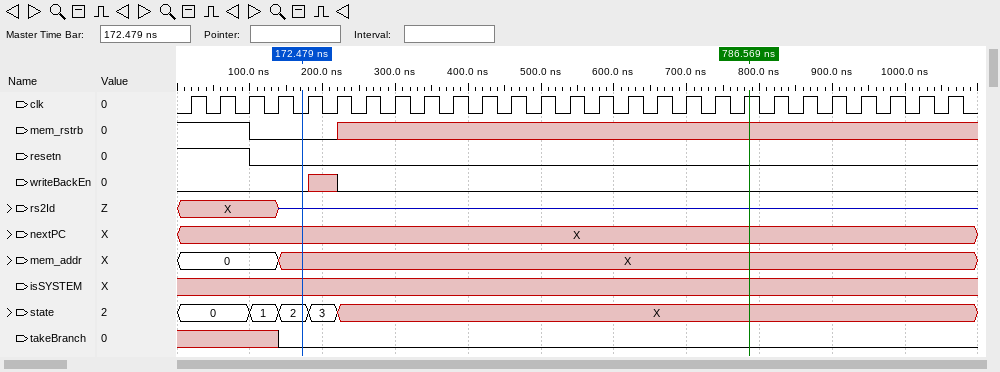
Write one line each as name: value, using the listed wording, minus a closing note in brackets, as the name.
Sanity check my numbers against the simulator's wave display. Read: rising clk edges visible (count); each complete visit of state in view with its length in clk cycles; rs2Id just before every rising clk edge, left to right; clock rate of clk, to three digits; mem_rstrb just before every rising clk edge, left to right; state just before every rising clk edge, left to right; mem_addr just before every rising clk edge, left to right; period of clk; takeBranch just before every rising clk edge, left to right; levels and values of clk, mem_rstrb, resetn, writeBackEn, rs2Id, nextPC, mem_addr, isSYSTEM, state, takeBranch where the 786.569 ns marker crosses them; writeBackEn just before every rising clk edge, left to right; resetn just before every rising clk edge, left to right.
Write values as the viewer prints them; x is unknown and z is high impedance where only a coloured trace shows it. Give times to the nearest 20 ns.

rising clk edges visible: 27
each complete visit of state in view with its length in clk cycles: 1: 1, 2: 1, 3: 1
rs2Id just before every rising clk edge, left to right: X, X, X, X, z, z, z, z, z, z, z, z, z, z, z, z, z, z, z, z, z, z, z, z, z, z, z
clock rate of clk, to three digits: 25.0 MHz
mem_rstrb just before every rising clk edge, left to right: 1 1 1 0 0 0 x x x x x x x x x x x x x x x x x x x x x
state just before every rising clk edge, left to right: 0, 0, 0, 1, 2, 3, X, X, X, X, X, X, X, X, X, X, X, X, X, X, X, X, X, X, X, X, X
mem_addr just before every rising clk edge, left to right: 0, 0, 0, 0, X, X, X, X, X, X, X, X, X, X, X, X, X, X, X, X, X, X, X, X, X, X, X
period of clk: 40 ns
takeBranch just before every rising clk edge, left to right: x x x x 0 0 0 0 0 0 0 0 0 0 0 0 0 0 0 0 0 0 0 0 0 0 0
levels and values of clk, mem_rstrb, resetn, writeBackEn, rs2Id, nextPC, mem_addr, isSYSTEM, state, takeBranch where the 786.569 ns marker crosses them: clk=1, mem_rstrb=x, resetn=0, writeBackEn=0, rs2Id=z, nextPC=X, mem_addr=X, isSYSTEM=x, state=X, takeBranch=0
writeBackEn just before every rising clk edge, left to right: 0 0 0 0 0 x 0 0 0 0 0 0 0 0 0 0 0 0 0 0 0 0 0 0 0 0 0
resetn just before every rising clk edge, left to right: 1 1 1 0 0 0 0 0 0 0 0 0 0 0 0 0 0 0 0 0 0 0 0 0 0 0 0
